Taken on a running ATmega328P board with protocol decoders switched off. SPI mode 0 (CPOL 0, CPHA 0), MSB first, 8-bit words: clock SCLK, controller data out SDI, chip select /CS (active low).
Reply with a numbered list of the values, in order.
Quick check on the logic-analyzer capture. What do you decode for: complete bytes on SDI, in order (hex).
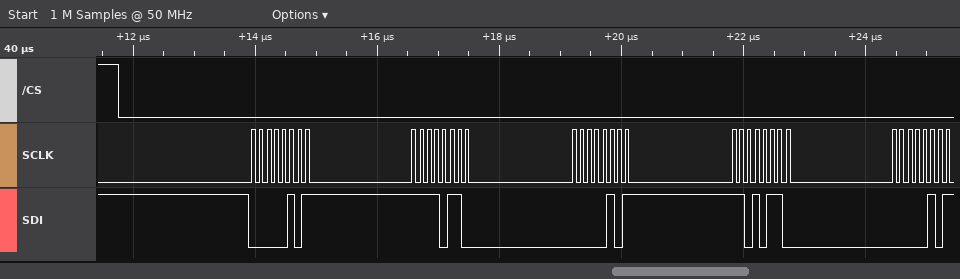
1. 05 F6 05 D6 05
